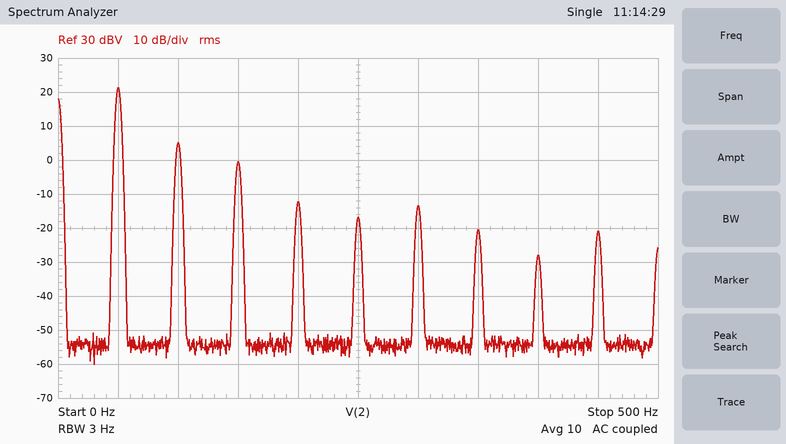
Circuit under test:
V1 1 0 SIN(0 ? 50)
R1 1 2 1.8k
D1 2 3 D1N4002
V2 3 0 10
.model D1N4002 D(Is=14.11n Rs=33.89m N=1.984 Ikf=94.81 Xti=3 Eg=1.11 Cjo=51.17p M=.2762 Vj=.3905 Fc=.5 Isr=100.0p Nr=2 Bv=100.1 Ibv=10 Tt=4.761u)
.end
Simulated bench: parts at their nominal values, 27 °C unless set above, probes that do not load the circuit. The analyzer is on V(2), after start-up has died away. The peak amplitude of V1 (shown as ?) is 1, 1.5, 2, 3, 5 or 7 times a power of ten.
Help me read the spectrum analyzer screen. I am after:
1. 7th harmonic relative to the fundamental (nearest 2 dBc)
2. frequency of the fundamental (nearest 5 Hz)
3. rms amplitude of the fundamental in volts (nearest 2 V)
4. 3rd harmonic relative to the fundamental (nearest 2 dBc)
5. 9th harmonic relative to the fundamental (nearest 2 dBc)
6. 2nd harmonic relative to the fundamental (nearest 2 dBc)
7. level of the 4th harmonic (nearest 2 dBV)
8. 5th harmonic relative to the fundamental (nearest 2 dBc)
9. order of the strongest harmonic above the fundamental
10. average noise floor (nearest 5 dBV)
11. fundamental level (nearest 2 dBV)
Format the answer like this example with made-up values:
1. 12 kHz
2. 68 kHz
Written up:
1. -42 dBc
2. 50 Hz
3. 12 V
4. -22 dBc
5. -42 dBc
6. -16 dBc
7. -12 dBV
8. -38 dBc
9. 2
10. -55 dBV
11. 22 dBV
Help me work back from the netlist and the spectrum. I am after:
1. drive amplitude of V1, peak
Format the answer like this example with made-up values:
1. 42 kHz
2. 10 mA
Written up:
1. 20 V
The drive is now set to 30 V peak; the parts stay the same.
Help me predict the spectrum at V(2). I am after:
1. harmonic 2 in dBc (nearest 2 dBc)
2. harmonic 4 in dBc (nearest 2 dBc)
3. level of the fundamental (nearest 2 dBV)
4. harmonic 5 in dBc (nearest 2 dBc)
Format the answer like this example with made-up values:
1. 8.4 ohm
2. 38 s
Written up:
1. -12 dBc
2. -38 dBc
3. 24 dBV
4. -30 dBc
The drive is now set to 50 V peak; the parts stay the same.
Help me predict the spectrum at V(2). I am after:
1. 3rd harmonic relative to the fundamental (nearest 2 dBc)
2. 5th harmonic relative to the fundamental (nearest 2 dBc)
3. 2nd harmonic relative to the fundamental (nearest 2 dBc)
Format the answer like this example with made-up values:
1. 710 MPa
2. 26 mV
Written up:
1. -24 dBc
2. -30 dBc
3. -10 dBc
